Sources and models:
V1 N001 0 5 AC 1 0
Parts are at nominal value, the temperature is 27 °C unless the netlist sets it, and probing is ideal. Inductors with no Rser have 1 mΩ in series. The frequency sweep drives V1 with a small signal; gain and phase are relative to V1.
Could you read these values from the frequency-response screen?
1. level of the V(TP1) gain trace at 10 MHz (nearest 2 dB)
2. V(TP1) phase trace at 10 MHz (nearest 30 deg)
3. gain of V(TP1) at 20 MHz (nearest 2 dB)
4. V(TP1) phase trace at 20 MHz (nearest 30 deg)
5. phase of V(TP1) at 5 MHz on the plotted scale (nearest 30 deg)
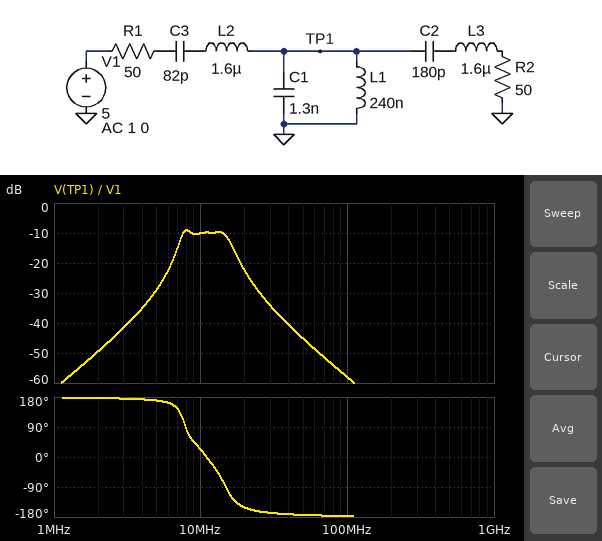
-10 dB
30 deg
-22 dB
-150 deg
180 deg
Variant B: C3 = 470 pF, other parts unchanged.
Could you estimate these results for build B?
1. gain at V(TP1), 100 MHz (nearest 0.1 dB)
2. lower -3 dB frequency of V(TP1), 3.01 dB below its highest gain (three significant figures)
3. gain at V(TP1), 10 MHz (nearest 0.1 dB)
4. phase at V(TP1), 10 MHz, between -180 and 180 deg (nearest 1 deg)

-58.2 dB
6.10 MHz
-6.8 dB
-56 deg
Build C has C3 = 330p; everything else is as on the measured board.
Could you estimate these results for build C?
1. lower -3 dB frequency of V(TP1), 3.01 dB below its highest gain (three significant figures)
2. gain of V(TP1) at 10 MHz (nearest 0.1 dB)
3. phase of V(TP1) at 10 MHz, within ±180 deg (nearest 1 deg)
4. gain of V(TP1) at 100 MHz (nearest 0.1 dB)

6.04 MHz
-6.3 dB
-48 deg
-58.2 dB
